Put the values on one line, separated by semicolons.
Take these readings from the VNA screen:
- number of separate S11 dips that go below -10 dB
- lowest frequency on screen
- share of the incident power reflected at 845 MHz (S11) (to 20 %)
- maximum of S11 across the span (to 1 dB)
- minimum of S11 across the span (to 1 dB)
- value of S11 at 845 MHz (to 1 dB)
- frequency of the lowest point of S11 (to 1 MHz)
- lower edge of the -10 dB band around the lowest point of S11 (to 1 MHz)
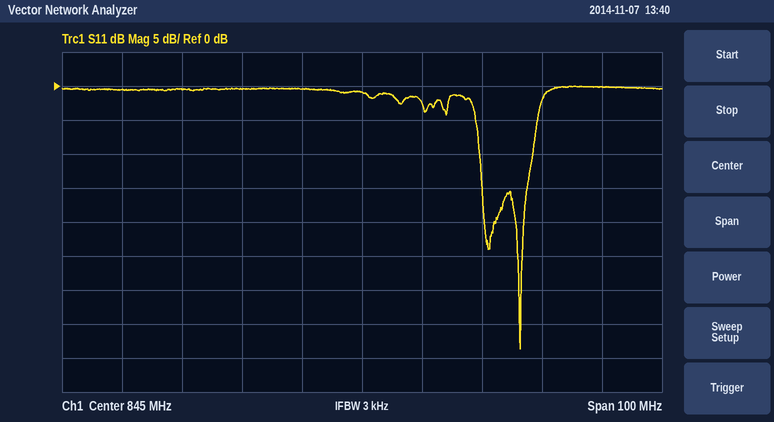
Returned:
2; 795 MHz; 80 %; 0 dB; -39 dB; -1 dB; 871 MHz; 865 MHz
